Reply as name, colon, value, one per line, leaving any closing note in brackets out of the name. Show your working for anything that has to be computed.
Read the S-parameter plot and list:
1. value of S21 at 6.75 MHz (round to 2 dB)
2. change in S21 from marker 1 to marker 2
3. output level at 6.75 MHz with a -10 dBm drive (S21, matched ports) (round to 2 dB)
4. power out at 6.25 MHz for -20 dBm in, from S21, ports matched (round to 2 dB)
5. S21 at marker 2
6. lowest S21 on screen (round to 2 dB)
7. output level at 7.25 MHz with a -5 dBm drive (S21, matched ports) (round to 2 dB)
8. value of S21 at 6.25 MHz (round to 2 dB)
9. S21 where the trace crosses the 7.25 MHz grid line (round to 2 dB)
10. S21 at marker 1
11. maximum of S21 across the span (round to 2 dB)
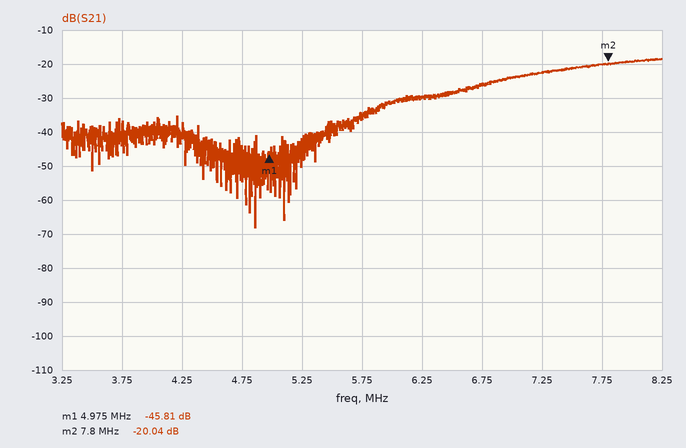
value of S21 at 6.75 MHz: -26 dB
change in S21 from marker 1 to marker 2: -20.04 − (-45.81) = 25.77 dB
output level at 6.75 MHz with a -10 dBm drive (S21, matched ports): -10 dBm + (-26 dB) = -36 dBm
power out at 6.25 MHz for -20 dBm in, from S21, ports matched: -20 dBm + (-30 dB) = -50 dBm
S21 at marker 2: -20.04 dB
lowest S21 on screen: -68 dB
output level at 7.25 MHz with a -5 dBm drive (S21, matched ports): -5 dBm + (-22 dB) = -28 dBm
value of S21 at 6.25 MHz: -30 dB
S21 where the trace crosses the 7.25 MHz grid line: -22 dB
S21 at marker 1: -45.81 dB
maximum of S21 across the span: -18 dB
